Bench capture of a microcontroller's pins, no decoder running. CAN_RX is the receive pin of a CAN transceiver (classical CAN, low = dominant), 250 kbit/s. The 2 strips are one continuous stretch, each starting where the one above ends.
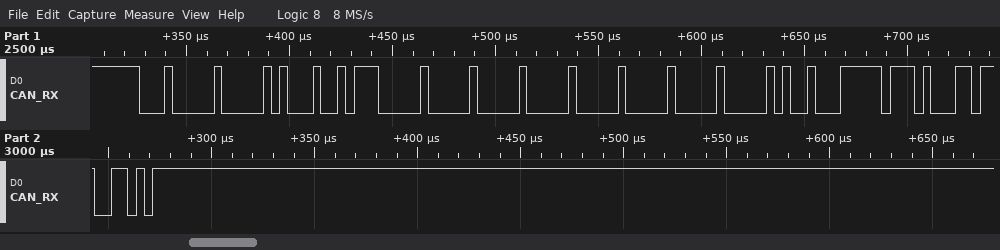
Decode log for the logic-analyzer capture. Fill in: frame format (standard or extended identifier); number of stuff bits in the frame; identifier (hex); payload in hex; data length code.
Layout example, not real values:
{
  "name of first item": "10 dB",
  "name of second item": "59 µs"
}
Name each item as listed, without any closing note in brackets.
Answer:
{
  "frame format": "standard",
  "number of stuff bits in the frame": "11",
  "identifier": "0x100",
  "payload in hex": "97 00 00 00 00 00 48 FF",
  "data length code": "8"
}
